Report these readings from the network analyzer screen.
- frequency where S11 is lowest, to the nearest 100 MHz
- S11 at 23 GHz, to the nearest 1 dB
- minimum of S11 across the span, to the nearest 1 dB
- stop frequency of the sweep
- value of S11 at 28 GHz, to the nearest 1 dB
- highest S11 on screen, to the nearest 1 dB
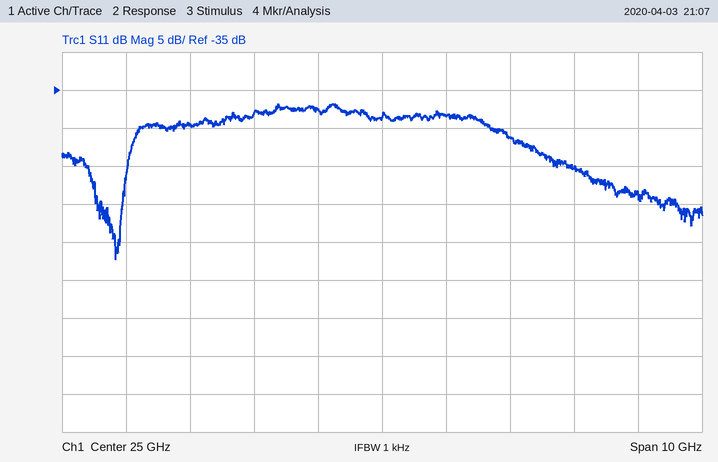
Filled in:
20.8 GHz
-38 dB
-57 dB
30 GHz
-45 dB
-37 dB
